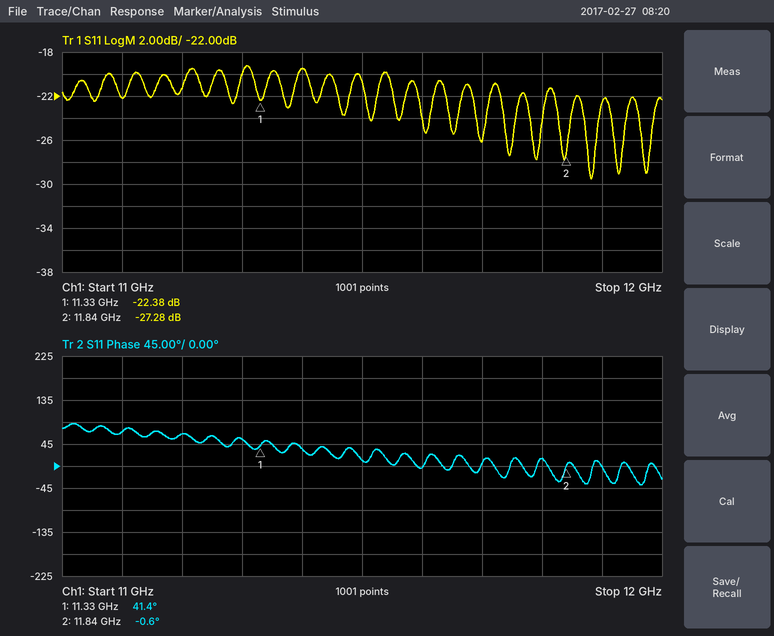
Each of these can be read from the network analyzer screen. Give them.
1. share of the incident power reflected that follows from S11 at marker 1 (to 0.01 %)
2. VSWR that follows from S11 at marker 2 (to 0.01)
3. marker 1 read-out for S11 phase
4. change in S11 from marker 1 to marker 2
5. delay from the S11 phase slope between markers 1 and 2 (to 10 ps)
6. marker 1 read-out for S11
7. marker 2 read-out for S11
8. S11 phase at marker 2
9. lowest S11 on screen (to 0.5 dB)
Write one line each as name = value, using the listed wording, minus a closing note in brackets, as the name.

share of the incident power reflected that follows from S11 at marker 1 = 0.58 %
VSWR that follows from S11 at marker 2 = 1.09
marker 1 read-out for S11 phase = 41.4°
change in S11 from marker 1 to marker 2 = -4.90 dB
delay from the S11 phase slope between markers 1 and 2 = 230 ps
marker 1 read-out for S11 = -22.38 dB
marker 2 read-out for S11 = -27.28 dB
S11 phase at marker 2 = -0.6°
lowest S11 on screen = -29.5 dB
